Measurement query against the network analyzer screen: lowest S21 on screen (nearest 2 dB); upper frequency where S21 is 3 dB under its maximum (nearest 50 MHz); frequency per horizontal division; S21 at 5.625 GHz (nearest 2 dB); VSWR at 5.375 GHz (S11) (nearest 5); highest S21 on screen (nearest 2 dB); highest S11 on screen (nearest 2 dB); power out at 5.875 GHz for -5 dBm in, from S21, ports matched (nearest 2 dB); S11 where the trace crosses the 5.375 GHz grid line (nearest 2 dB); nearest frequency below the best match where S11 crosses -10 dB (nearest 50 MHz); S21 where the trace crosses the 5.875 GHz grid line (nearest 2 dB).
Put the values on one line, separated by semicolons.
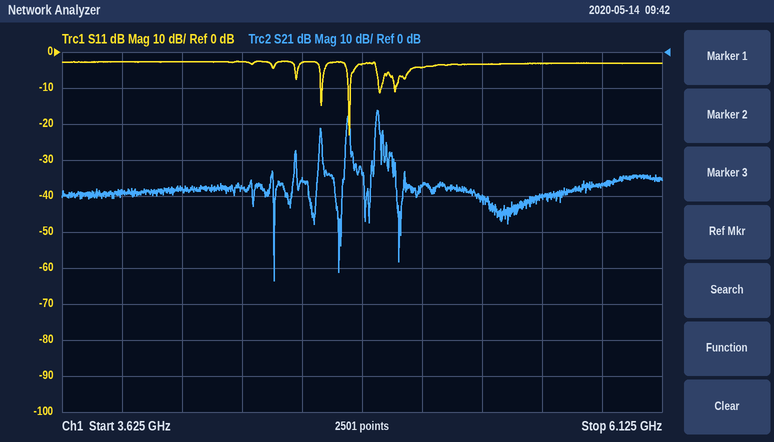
-64 dB; 4.95 GHz; 250 MHz; -40 dB; 5; -16 dB; -2 dB; -42 dBm; -4 dB; 4.80 GHz; -36 dB
